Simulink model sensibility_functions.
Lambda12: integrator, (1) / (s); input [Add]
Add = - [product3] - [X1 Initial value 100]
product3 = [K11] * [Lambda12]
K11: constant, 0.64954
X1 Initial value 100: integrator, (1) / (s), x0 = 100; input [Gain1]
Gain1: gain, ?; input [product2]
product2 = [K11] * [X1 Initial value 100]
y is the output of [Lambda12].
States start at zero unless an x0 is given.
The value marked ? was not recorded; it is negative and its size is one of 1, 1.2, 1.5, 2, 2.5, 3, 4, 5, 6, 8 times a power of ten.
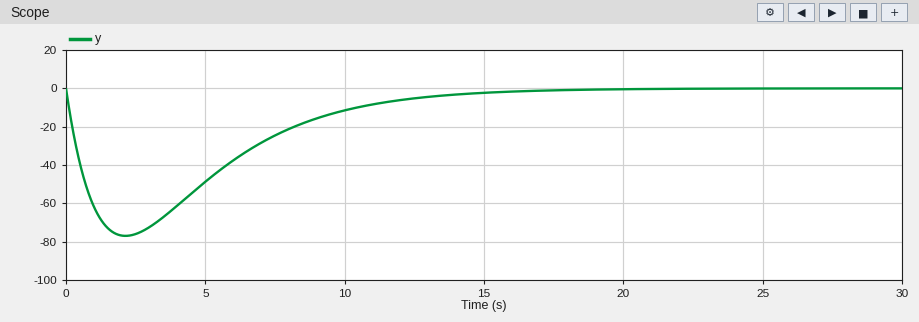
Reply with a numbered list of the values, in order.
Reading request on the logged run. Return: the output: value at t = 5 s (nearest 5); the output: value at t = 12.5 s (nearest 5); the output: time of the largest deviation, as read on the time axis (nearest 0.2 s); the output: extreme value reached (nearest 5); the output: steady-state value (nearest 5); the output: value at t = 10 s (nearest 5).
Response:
1. -50
2. -5
3. 2.2 s
4. -75
5. 0
6. -10
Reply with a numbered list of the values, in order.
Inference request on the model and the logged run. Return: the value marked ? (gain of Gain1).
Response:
1. -0.5
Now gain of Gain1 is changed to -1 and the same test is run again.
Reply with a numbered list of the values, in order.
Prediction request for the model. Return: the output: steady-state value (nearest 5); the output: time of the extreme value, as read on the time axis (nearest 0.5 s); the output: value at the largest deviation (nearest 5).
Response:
1. 0
2. 1.5 s
3. -55
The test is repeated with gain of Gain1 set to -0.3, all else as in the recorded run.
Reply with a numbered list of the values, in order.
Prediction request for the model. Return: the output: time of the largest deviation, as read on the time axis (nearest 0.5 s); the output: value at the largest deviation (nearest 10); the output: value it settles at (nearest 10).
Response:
1. 2.5 s
2. -90
3. 0
